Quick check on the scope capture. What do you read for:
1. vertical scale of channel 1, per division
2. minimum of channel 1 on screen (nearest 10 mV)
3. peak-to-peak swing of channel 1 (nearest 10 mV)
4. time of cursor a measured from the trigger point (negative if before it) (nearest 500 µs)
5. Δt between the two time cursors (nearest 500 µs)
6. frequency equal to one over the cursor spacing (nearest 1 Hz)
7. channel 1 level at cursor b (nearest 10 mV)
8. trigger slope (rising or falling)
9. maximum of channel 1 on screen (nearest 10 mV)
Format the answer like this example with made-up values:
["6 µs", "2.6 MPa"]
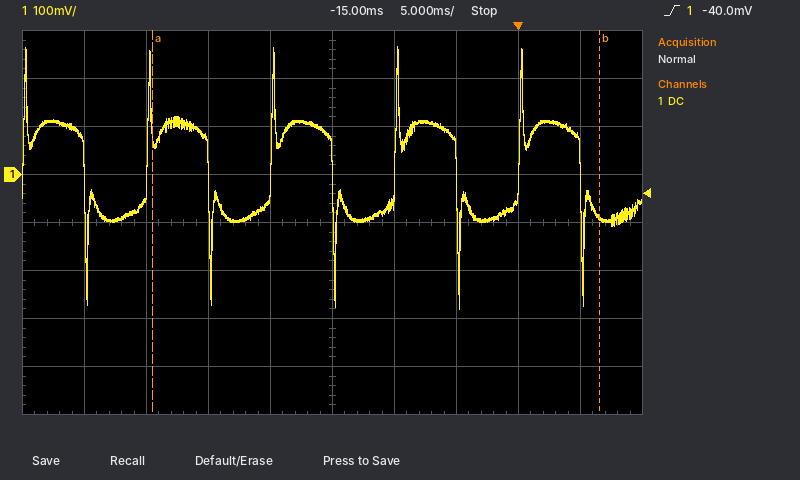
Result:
["100 mV", "-280 mV", "550 mV", "-29.5 ms", "36.0 ms", "28 Hz", "-90 mV", "rising", "270 mV"]
